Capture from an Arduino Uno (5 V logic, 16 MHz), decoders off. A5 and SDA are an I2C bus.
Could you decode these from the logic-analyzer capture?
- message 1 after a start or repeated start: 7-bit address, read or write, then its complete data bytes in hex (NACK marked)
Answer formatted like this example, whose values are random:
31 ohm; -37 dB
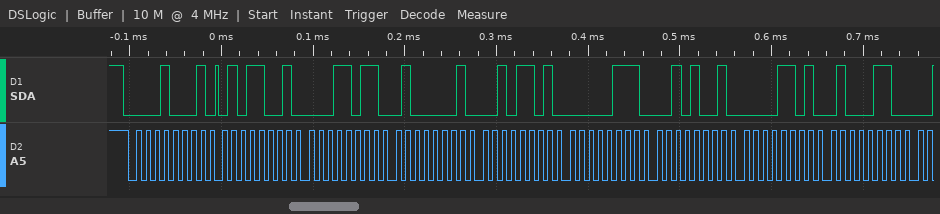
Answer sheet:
0x08 read: 59 1B 41 2D 07 29 0D 46
